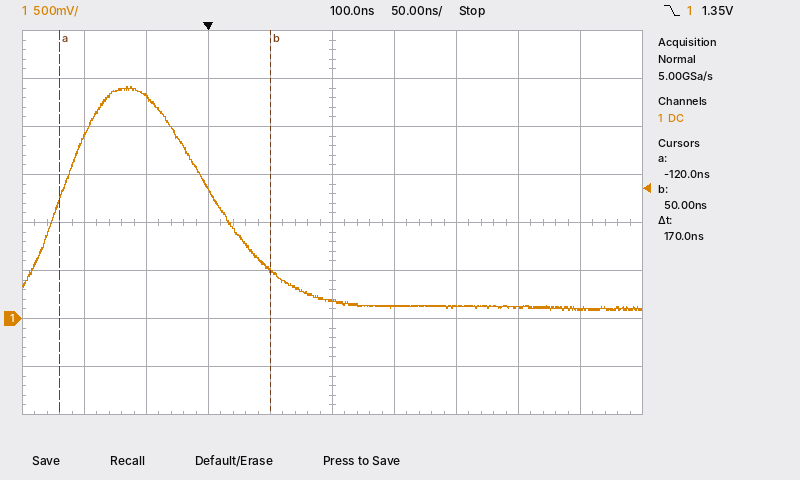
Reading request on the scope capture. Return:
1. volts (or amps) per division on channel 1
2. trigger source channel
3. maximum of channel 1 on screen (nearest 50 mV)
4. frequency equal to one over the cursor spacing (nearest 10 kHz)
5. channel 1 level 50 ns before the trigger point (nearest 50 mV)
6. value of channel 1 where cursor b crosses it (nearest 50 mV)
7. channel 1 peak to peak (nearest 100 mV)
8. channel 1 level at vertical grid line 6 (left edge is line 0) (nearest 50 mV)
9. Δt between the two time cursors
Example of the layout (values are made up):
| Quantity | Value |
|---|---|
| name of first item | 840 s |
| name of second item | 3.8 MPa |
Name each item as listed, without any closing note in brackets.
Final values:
| Quantity | Value |
|---|---|
| volts (or amps) per division on channel 1 | 500 mV |
| trigger source channel | channel 1 |
| maximum of channel 1 on screen | 2.40 V |
| frequency equal to one over the cursor spacing | 5.88 MHz |
| channel 1 level 50 ns before the trigger point | 2.30 V |
| value of channel 1 where cursor b crosses it | 500 mV |
| channel 1 peak to peak | 2.30 V |
| channel 1 level at vertical grid line 6 (left edge is line 0) | 150 mV |
| Δt between the two time cursors | 170 ns |
